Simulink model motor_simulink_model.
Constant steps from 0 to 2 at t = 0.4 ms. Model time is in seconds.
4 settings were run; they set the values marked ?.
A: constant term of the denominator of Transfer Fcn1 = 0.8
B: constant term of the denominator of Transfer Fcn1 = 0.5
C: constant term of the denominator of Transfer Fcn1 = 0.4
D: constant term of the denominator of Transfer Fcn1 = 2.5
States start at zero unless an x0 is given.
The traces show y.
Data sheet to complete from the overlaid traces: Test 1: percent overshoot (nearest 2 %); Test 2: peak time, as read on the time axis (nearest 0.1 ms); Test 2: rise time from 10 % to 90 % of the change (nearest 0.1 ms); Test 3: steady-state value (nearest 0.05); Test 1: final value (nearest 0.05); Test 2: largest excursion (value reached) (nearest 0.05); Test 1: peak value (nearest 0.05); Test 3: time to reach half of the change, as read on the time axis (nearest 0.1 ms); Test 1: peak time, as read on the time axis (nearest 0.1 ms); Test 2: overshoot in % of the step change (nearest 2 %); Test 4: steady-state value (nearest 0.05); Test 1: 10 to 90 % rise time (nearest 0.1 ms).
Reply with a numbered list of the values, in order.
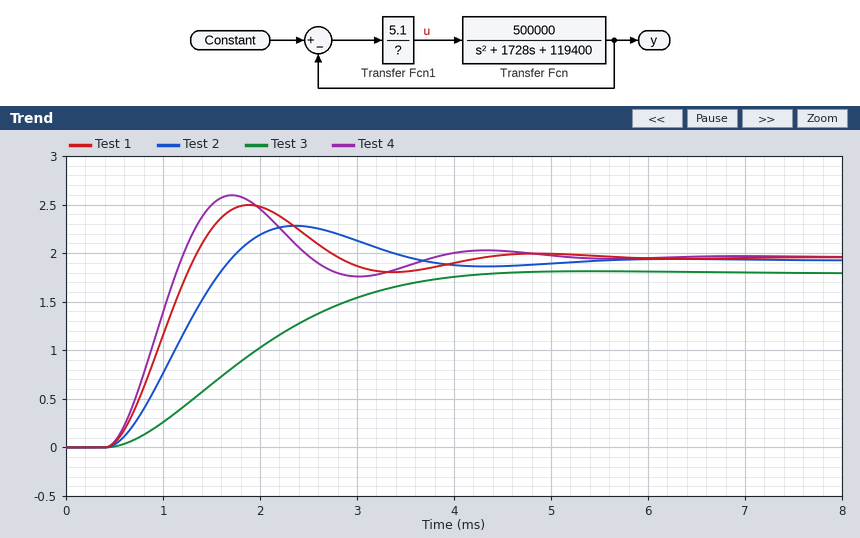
1. 28 %
2. 2.4 ms
3. 0.9 ms
4. 1.80
5. 1.95
6. 2.30
7. 2.50
8. 1.8 ms
9. 1.9 ms
10. 18 %
11. 1.95
12. 0.6 ms
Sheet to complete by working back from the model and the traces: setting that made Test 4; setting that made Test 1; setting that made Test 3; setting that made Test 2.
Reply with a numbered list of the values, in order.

1. C
2. B
3. D
4. A
